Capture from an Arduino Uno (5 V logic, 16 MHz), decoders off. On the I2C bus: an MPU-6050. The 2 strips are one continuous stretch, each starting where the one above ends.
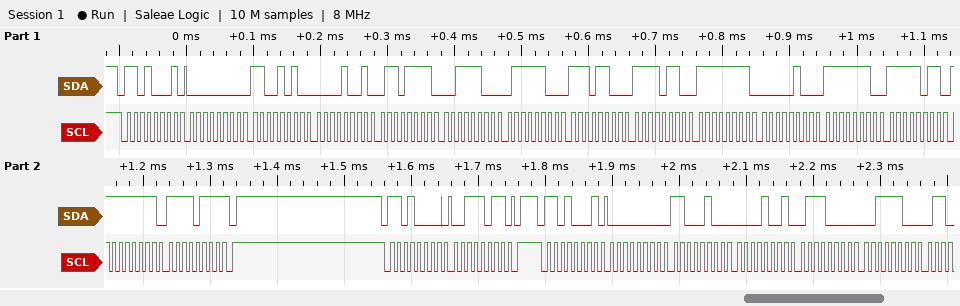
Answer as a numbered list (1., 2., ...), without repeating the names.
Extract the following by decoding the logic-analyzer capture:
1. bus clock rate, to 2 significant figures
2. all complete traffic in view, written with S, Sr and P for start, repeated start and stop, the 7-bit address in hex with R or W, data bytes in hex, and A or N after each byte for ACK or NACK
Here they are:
1. 100 kHz
2. S 68R A 00 A CA A 09 A 6F A 3C A 7C A EC A F6 A FF A 04 A FE A FB A FF A F7 N P S 68W A 3B A P S 68R A 00 A C4 A 09 A 70 A 3C A
